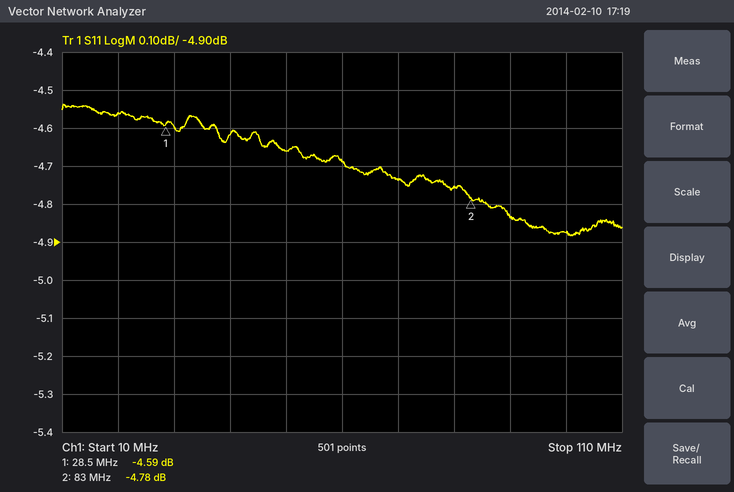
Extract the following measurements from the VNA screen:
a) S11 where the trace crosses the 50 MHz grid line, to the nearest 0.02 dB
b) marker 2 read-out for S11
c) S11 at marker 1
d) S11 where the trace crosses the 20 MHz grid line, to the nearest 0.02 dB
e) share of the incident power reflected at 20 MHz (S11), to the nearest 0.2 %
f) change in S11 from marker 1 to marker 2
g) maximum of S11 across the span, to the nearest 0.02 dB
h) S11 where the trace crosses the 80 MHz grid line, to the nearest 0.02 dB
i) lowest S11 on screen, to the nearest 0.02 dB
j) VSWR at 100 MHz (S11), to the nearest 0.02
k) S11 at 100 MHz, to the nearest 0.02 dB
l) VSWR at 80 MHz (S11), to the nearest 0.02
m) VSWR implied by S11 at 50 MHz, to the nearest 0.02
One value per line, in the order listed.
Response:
-4.66 dB
-4.78 dB
-4.59 dB
-4.56 dB
35.0 %
-0.19 dB
-4.54 dB
-4.76 dB
-4.88 dB
3.66
-4.88 dB
3.74
3.82
